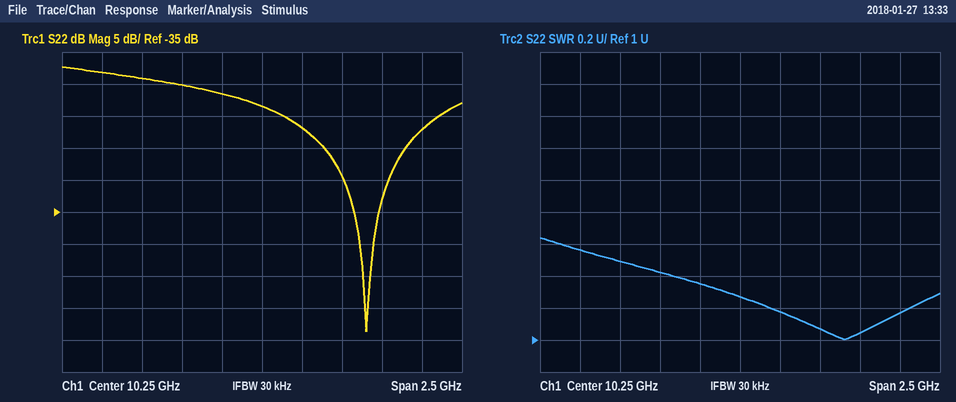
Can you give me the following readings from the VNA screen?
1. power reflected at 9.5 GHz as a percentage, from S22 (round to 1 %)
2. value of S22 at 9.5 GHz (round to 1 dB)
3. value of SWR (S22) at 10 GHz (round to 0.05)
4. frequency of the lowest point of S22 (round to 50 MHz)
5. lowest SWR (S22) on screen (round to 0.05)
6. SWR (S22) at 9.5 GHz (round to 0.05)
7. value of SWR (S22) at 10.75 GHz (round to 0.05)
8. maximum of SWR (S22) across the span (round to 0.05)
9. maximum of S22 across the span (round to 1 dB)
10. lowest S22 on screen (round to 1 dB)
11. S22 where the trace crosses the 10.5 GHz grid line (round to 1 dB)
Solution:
4 %
-14 dB
1.35
10.90 GHz
1.00
1.50
1.05
1.65
-12 dB
-54 dB
-22 dB
